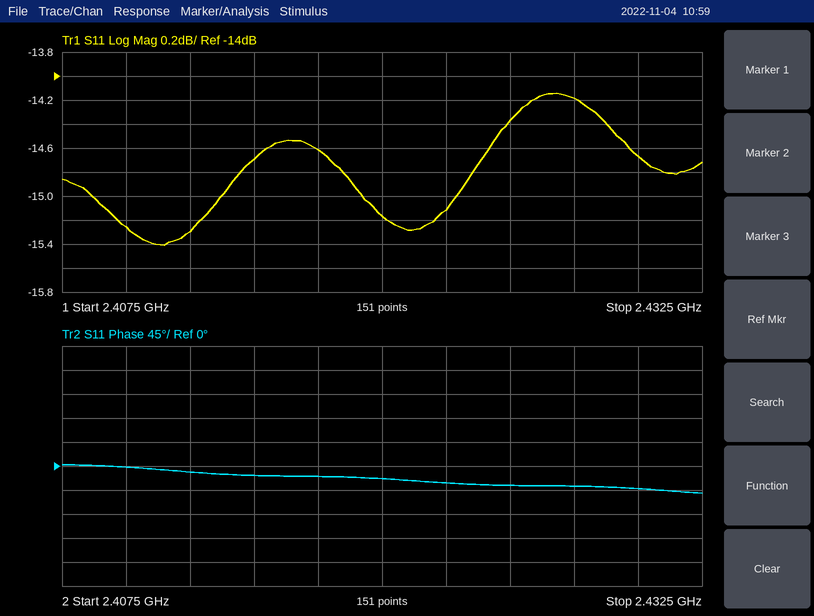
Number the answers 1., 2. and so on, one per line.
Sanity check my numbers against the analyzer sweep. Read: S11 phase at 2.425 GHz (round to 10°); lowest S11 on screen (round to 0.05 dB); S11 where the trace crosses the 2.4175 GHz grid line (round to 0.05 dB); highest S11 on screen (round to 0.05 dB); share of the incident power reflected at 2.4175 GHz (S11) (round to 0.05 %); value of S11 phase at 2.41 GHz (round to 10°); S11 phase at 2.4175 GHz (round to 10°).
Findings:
1. -40°
2. -15.40 dB
3. -14.60 dB
4. -14.15 dB
5. 3.45 %
6. 0°
7. -20°
